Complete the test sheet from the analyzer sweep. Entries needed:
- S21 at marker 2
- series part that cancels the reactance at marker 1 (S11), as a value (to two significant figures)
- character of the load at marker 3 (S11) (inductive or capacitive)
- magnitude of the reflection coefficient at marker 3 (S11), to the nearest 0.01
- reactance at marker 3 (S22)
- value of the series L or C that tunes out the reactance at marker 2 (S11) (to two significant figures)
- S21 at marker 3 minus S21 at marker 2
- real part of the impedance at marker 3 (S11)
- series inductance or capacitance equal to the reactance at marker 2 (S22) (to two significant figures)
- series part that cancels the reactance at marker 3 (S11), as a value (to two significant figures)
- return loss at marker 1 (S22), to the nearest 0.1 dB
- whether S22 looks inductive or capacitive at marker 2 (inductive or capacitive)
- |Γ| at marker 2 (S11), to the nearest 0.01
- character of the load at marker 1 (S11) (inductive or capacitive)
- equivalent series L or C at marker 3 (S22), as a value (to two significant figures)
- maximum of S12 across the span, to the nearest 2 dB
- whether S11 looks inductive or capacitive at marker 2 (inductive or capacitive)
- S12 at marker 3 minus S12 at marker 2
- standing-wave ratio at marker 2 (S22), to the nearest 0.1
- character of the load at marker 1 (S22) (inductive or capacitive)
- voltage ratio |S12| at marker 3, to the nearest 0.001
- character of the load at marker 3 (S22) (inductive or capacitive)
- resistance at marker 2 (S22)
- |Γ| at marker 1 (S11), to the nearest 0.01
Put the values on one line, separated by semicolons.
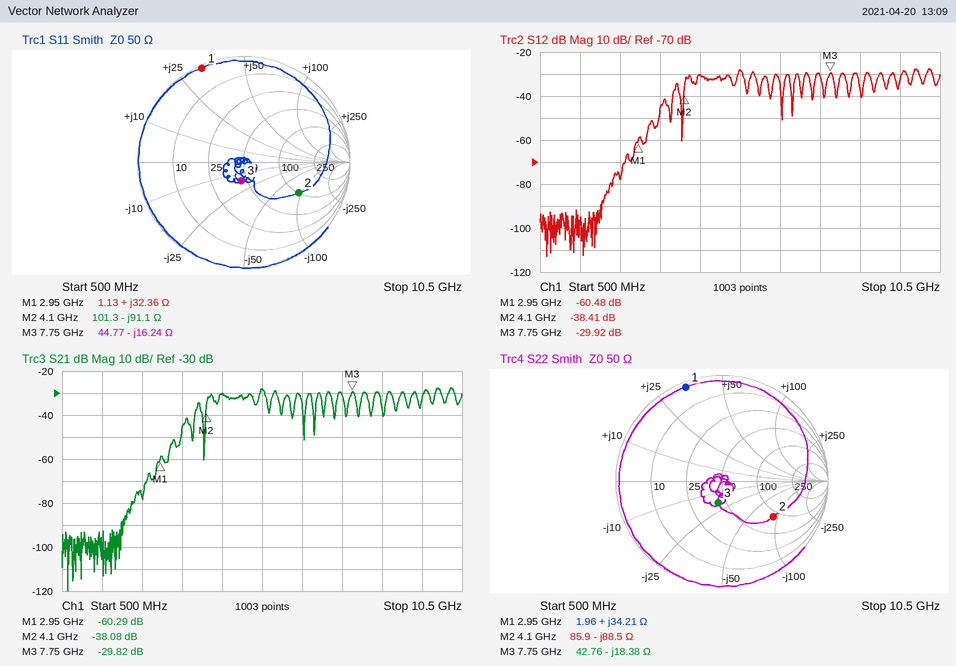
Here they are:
-38.08 dB; 1.7 pF; capacitive; 0.18; -18.38 Ω; 3.5 nH; 8.26 dB; 44.77 Ω; 440 fF; 330 pH; 0.5 dB; capacitive; 0.59; inductive; 1.1 pF; -28 dB; capacitive; 8.49 dB; 3.9; inductive; 0.032; capacitive; 85.9 Ω; 0.97
